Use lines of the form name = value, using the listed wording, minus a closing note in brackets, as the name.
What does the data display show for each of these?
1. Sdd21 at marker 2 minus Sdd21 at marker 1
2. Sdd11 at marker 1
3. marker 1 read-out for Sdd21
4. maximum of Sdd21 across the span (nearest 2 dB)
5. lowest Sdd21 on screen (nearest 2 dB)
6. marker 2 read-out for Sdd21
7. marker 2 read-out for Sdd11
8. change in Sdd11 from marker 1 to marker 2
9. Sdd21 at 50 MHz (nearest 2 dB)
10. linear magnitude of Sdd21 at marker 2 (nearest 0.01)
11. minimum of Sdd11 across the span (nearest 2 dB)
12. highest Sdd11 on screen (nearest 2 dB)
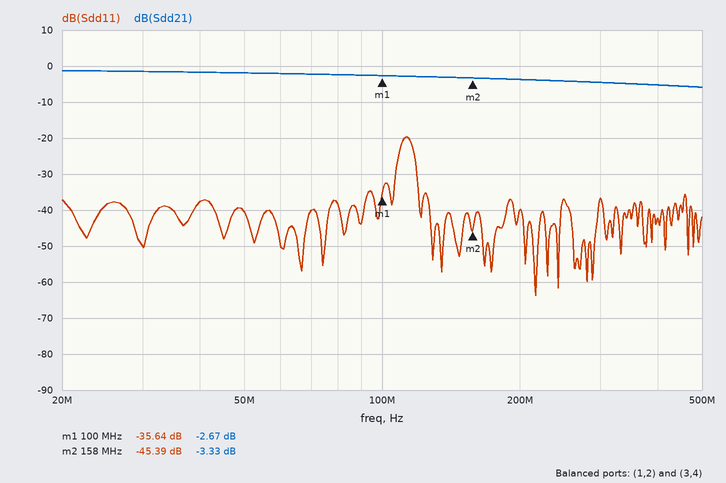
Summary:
Sdd21 at marker 2 minus Sdd21 at marker 1 = -0.66 dB
Sdd11 at marker 1 = -35.64 dB
marker 1 read-out for Sdd21 = -2.67 dB
maximum of Sdd21 across the span = -2 dB
lowest Sdd21 on screen = -6 dB
marker 2 read-out for Sdd21 = -3.33 dB
marker 2 read-out for Sdd11 = -45.39 dB
change in Sdd11 from marker 1 to marker 2 = -9.75 dB
Sdd21 at 50 MHz = -2 dB
linear magnitude of Sdd21 at marker 2 = 0.68
minimum of Sdd11 across the span = -64 dB
highest Sdd11 on screen = -20 dB
